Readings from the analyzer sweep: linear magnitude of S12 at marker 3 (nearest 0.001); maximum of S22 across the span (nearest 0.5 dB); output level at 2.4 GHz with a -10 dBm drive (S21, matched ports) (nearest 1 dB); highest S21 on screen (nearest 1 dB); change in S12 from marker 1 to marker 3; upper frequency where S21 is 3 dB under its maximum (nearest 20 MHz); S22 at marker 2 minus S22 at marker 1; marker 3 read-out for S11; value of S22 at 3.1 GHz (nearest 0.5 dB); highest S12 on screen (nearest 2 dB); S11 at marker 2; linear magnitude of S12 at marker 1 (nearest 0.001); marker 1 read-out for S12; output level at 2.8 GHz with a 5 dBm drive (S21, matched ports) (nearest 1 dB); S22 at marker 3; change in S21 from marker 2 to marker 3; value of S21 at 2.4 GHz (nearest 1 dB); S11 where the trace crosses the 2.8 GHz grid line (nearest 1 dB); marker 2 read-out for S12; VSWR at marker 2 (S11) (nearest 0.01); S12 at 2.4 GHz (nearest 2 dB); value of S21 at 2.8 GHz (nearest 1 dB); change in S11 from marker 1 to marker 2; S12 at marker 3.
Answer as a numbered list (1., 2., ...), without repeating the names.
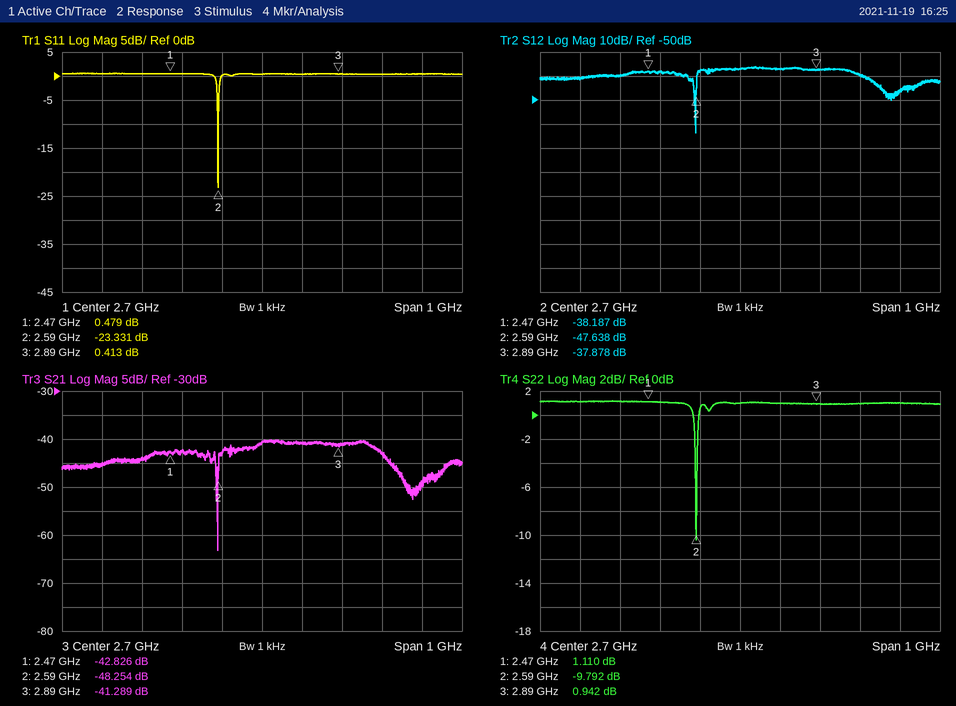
1. 0.013
2. 1.0 dB
3. -54 dBm
4. -40 dB
5. 0.309 dB
6. 3.00 GHz
7. -10.902 dB
8. 0.413 dB
9. 1.0 dB
10. -36 dB
11. -23.331 dB
12. 0.012
13. -38.187 dB
14. -36 dBm
15. 0.942 dB
16. 6.965 dB
17. -44 dB
18. 0 dB
19. -47.638 dB
20. 1.15
21. -40 dB
22. -41 dB
23. -23.810 dB
24. -37.878 dB
